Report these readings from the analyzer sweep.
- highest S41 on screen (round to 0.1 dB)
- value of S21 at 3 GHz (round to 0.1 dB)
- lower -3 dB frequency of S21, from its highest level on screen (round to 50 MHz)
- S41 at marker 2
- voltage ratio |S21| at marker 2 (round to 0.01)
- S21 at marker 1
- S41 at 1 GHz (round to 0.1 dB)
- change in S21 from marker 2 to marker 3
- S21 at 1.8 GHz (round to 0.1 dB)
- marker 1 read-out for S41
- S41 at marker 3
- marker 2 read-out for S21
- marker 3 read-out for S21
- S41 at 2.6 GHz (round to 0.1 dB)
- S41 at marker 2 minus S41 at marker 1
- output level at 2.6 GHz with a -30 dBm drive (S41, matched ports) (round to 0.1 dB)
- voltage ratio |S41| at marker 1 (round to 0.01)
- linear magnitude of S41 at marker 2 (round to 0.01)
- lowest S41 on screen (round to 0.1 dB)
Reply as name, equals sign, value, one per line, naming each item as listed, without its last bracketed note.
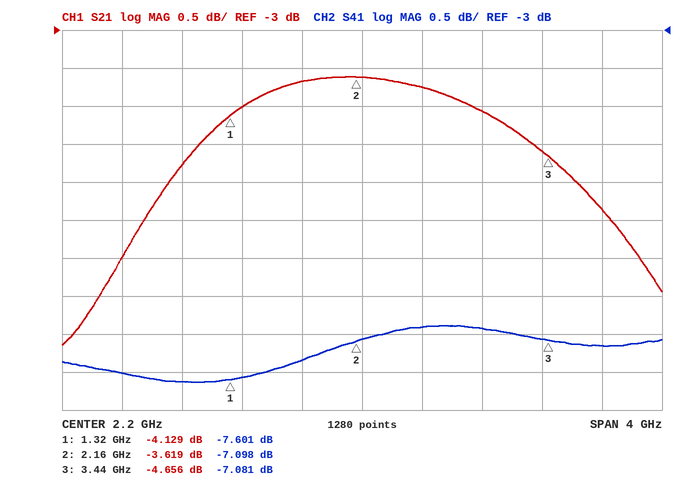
highest S41 on screen = -6.9 dB
value of S21 at 3 GHz = -4.1 dB
lower -3 dB frequency of S21, from its highest level on screen = 400 MHz
S41 at marker 2 = -7.098 dB
voltage ratio |S21| at marker 2 = 0.66
S21 at marker 1 = -4.129 dB
S41 at 1 GHz = -7.6 dB
change in S21 from marker 2 to marker 3 = -1.037 dB
S21 at 1.8 GHz = -3.7 dB
marker 1 read-out for S41 = -7.601 dB
S41 at marker 3 = -7.081 dB
marker 2 read-out for S21 = -3.619 dB
marker 3 read-out for S21 = -4.656 dB
S41 at 2.6 GHz = -6.9 dB
S41 at marker 2 minus S41 at marker 1 = 0.503 dB
output level at 2.6 GHz with a -30 dBm drive (S41, matched ports) = -36.9 dBm
voltage ratio |S41| at marker 1 = 0.42
linear magnitude of S41 at marker 2 = 0.44
lowest S41 on screen = -7.6 dB
